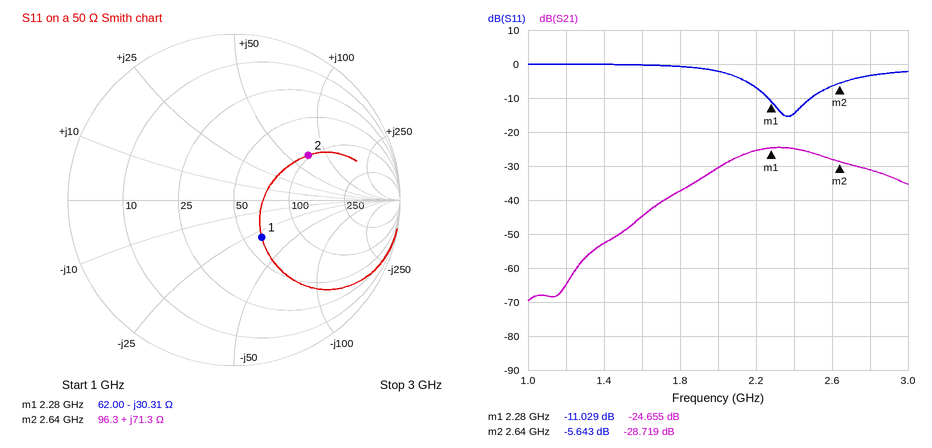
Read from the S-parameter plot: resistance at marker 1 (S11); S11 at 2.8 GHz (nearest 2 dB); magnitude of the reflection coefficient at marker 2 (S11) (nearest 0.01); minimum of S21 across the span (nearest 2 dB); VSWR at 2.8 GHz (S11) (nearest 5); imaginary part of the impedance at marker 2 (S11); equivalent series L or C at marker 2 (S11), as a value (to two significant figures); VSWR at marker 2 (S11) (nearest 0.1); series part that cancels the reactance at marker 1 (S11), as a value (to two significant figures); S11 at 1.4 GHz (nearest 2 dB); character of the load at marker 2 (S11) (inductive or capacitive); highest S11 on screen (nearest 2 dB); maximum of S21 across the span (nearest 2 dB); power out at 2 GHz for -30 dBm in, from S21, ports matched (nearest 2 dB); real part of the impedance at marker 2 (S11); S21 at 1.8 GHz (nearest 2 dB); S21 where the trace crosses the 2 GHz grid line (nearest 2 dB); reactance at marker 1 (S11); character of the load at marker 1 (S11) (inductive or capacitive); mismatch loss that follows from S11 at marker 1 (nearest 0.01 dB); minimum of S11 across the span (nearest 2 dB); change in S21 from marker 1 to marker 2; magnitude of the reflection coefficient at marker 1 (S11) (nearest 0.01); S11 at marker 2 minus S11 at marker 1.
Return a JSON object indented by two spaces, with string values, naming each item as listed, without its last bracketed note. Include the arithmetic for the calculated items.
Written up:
{
  "resistance at marker 1": "62.00 Ω",
  "S11 at 2.8 GHz": "-4 dB",
  "magnitude of the reflection coefficient at marker 2 (S11)": "0.52",
  "minimum of S21 across the span": "-70 dB",
  "VSWR at 2.8 GHz (S11)": "|Γ| = 10^(-4/20) = 0.6310; VSWR = (1 + 0.6310)/(1 − 0.6310) ≈ 4.42, so 5 to the nearest 5",
  "imaginary part of the impedance at marker 2": "+71.3 Ω",
  "equivalent series L or C at marker 2 (S11), as a value": "L = 71.3 Ω/(2π × 2.64 GHz) ≈ 4.3 nH",
  "VSWR at marker 2 (S11)": "(1 + 0.5222)/(1 − 0.5222) ≈ 3.2",
  "series part that cancels the reactance at marker 1 (S11), as a value": "L = 30.31 Ω/(2π × 2.28 GHz) ≈ 2.1 nH",
  "S11 at 1.4 GHz": "0 dB",
  "character of the load at marker 2 (S11)": "inductive",
  "highest S11 on screen": "0 dB",
  "maximum of S21 across the span": "-24 dB",
  "power out at 2 GHz for -30 dBm in, from S21, ports matched": "-30 dBm + (-30 dB) = -60 dBm",
  "real part of the impedance at marker 2": "96.3 Ω",
  "S21 at 1.8 GHz": "-38 dB",
  "S21 where the trace crosses the 2 GHz grid line": "-30 dB",
  "reactance at marker 1": "-30.31 Ω",
  "character of the load at marker 1 (S11)": "capacitive",
  "mismatch loss that follows from S11 at marker 1": "−10 log10(1 − 10^(-11.029/10)) ≈ 0.36 dB",
  "minimum of S11 across the span": "-16 dB",
  "change in S21 from marker 1 to marker 2": "-28.719 − (-24.655) = -4.064 dB",
  "magnitude of the reflection coefficient at marker 1 (S11)": "0.28",
  "S11 at marker 2 minus S11 at marker 1": "-5.643 − (-11.029) = 5.386 dB"
}
